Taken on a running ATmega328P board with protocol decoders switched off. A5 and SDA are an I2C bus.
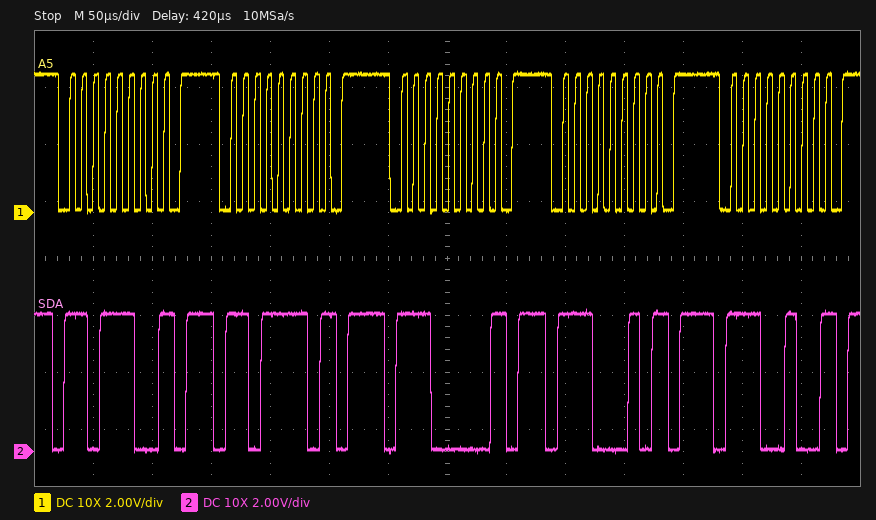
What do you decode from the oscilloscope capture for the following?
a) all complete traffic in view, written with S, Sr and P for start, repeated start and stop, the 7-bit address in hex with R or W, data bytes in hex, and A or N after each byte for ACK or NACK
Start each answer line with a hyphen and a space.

- S 6EW N P S 6FW N P S 70W N P S 71W N P S 72W N P
